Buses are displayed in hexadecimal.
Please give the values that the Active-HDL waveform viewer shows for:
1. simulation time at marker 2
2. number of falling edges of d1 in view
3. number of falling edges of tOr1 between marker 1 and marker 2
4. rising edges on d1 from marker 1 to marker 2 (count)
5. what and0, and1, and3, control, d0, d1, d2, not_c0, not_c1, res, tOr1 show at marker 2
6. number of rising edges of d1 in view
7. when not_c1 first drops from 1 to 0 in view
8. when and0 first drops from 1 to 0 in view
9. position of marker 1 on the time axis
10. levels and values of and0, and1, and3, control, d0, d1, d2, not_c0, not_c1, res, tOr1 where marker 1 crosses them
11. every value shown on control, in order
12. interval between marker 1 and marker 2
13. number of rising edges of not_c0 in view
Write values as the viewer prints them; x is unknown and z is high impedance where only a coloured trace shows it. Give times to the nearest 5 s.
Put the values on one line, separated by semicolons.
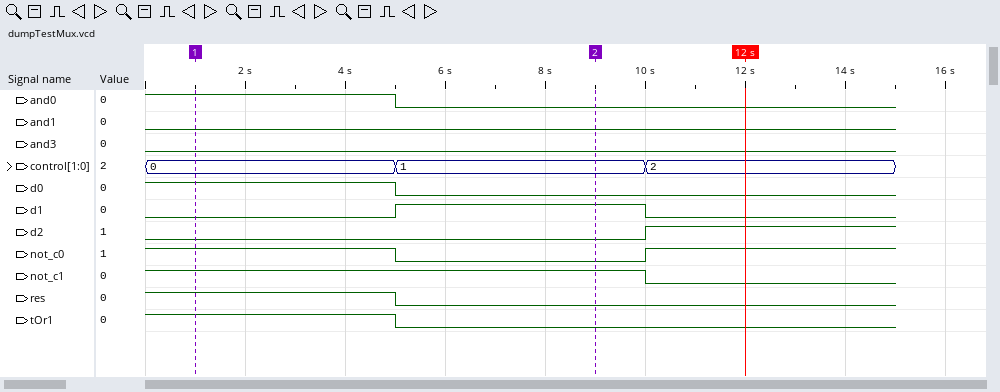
10 s; 1; 1; 1; and0=0, and1=0, and3=0, control=1, d0=0, d1=1, d2=0, not_c0=0, not_c1=1, res=0, tOr1=0; 1; 10 s; 5 s; 0 s; and0=1, and1=0, and3=0, control=0, d0=1, d1=0, d2=0, not_c0=1, not_c1=1, res=1, tOr1=1; 0, 1, 2; 10 s; 1
